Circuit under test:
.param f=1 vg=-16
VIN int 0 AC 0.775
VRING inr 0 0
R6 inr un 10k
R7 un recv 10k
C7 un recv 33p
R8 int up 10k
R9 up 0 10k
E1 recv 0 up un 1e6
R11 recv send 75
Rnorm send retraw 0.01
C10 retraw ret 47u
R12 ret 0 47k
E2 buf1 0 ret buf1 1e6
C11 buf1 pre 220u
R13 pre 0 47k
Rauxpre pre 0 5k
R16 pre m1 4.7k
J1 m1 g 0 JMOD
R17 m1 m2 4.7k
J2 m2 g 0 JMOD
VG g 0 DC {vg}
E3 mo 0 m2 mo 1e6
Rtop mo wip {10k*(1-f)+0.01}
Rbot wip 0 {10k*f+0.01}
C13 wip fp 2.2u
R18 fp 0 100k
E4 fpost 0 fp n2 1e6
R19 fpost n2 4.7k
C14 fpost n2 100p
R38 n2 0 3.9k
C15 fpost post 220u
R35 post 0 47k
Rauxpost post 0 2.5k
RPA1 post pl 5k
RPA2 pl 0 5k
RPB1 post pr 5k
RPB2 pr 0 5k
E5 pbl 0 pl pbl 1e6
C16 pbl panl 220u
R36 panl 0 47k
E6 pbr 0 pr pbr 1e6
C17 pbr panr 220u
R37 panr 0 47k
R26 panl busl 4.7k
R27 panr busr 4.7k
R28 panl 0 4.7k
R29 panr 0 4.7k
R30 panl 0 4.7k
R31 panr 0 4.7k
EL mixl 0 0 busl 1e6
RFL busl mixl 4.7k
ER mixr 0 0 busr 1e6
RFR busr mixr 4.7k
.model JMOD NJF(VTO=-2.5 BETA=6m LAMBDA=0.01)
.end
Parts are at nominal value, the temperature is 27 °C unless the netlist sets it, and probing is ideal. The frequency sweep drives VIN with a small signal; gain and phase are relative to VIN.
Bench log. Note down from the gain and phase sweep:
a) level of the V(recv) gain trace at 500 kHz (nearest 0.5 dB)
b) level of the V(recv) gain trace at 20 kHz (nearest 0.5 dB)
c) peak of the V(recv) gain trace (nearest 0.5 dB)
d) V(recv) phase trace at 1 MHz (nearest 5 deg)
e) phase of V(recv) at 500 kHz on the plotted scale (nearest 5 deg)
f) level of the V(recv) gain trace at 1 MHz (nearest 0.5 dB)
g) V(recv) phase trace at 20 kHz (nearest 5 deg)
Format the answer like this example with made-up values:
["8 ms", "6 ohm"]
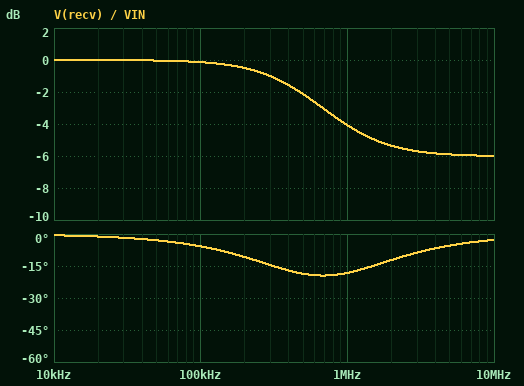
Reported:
["-2.0 dB", "0 dB", "0 dB", "-20 deg", "-20 deg", "-4.0 dB", "0 deg"]
